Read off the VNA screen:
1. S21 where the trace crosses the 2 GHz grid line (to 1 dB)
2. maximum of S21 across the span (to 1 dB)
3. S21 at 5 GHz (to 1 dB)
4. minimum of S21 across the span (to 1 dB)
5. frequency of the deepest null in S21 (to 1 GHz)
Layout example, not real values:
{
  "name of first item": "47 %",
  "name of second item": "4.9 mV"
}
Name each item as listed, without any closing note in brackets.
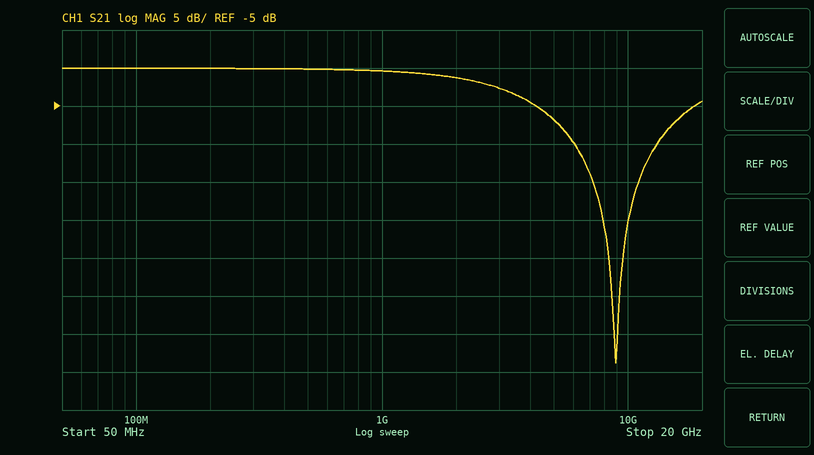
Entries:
{
  "S21 where the trace crosses the 2 GHz grid line": "-1 dB",
  "maximum of S21 across the span": "0 dB",
  "S21 at 5 GHz": "-7 dB",
  "minimum of S21 across the span": "-39 dB",
  "frequency of the deepest null in S21": "9 GHz"
}
